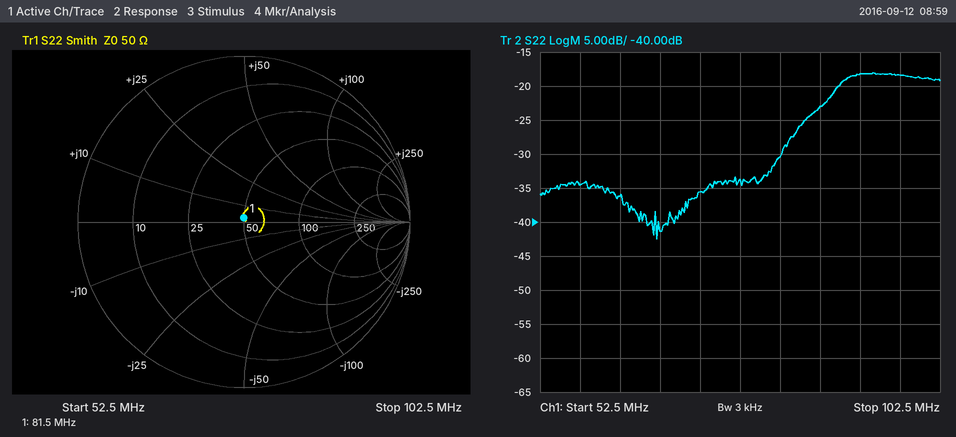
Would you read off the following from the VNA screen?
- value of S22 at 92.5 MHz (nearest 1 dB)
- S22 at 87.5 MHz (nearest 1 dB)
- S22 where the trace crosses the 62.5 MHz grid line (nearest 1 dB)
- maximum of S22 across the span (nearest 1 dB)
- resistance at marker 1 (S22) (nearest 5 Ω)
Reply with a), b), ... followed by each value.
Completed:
a) -18 dB
b) -23 dB
c) -36 dB
d) -18 dB
e) 50 Ω
